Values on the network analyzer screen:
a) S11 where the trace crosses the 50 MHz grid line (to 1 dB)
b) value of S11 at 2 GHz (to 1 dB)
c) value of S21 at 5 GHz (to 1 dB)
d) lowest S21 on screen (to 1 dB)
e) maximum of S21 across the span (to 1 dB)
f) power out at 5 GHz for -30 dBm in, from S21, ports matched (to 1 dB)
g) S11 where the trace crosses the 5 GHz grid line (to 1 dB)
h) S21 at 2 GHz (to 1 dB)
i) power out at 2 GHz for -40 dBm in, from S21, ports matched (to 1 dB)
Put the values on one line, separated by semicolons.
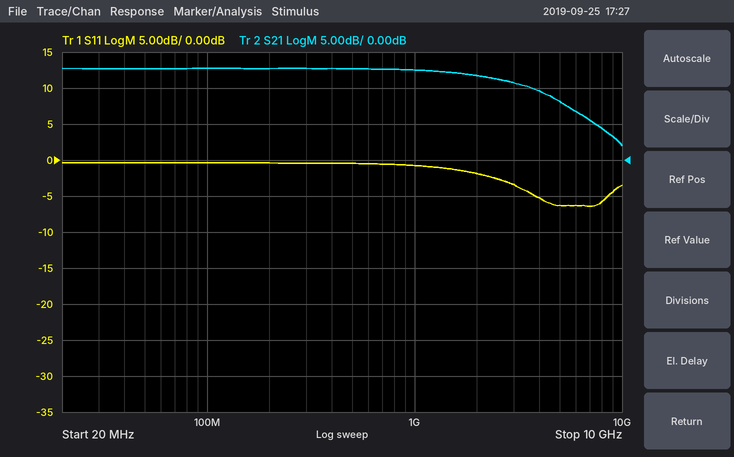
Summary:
0 dB; -2 dB; 8 dB; 2 dB; 13 dB; -22 dBm; -6 dB; 12 dB; -28 dBm
